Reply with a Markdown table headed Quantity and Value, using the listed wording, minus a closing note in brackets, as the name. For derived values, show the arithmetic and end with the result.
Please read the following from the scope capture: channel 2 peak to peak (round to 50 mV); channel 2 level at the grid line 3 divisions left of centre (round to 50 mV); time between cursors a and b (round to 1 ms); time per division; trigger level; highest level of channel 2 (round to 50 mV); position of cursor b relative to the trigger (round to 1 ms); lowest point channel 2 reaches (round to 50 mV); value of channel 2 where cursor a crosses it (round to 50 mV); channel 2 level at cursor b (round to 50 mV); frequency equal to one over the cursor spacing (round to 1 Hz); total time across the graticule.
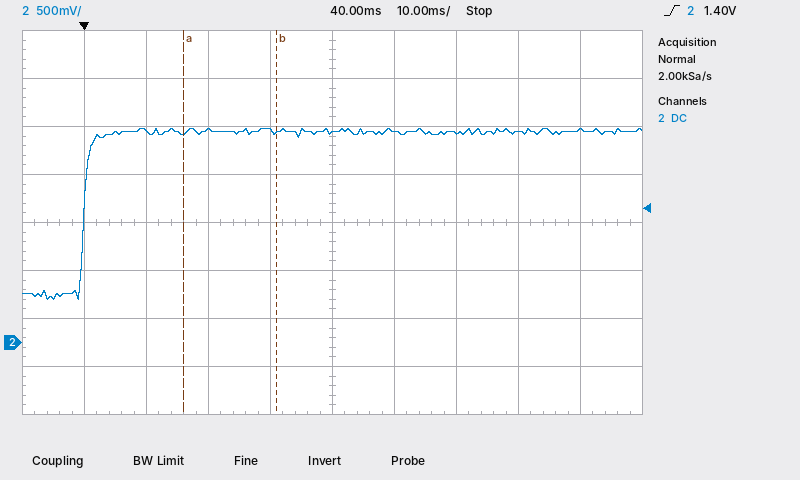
| Quantity | Value |
|---|---|
| channel 2 peak to peak | 2.25 V − (450 mV) = 1.80 V |
| channel 2 level at the grid line 3 divisions left of centre | 2.20 V |
| time between cursors a and b | 15 ms |
| time per division | 10 ms |
| trigger level | 1.40 V |
| highest level of channel 2 | 2.25 V |
| position of cursor b relative to the trigger | +31 ms |
| lowest point channel 2 reaches | 450 mV |
| value of channel 2 where cursor a crosses it | 2.20 V |
| channel 2 level at cursor b | 2.20 V |
| frequency equal to one over the cursor spacing | 1 / 15 ms ≈ 67 Hz |
| total time across the graticule | 100 ms |
